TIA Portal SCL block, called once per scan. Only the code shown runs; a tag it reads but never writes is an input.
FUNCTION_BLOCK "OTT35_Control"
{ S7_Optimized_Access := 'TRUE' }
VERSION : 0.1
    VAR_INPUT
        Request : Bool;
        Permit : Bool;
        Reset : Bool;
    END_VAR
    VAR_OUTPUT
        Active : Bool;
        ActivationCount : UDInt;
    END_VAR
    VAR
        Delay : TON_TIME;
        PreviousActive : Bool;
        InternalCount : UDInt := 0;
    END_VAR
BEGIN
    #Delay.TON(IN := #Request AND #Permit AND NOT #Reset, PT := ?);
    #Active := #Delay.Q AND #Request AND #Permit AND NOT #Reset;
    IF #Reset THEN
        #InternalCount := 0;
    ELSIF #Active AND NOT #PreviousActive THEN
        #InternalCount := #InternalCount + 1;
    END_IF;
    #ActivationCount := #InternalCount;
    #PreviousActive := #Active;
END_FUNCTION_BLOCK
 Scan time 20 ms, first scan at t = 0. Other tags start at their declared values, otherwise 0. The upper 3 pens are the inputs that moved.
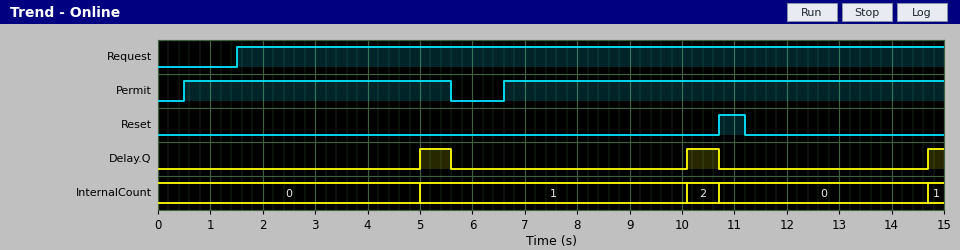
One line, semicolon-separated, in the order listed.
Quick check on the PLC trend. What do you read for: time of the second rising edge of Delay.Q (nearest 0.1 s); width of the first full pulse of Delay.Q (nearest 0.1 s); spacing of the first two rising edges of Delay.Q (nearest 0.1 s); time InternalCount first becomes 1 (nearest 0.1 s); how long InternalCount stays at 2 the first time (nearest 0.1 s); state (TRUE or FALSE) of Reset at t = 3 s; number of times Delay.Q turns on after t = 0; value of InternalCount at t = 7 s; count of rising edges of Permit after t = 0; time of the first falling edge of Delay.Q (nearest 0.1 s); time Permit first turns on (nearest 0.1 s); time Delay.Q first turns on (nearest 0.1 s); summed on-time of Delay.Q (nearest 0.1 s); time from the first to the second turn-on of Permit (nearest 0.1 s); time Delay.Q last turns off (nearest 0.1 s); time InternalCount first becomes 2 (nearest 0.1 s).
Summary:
10.1 s; 0.6 s; 5.1 s; 5.0 s; 0.6 s; FALSE; 3; 1; 2; 5.6 s; 0.5 s; 5.0 s; 1.5 s; 6.1 s; 10.7 s; 10.1 s
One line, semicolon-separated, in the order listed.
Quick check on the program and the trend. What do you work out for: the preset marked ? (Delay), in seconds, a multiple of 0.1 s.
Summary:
3.5 s
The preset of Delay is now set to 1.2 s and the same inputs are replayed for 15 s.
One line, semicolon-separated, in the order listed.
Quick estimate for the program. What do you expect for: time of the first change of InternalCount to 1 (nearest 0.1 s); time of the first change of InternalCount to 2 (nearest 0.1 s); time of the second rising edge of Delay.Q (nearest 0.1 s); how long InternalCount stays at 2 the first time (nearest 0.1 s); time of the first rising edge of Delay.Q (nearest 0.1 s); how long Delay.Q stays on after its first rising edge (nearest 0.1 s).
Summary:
2.7 s; 7.8 s; 7.8 s; 2.9 s; 2.7 s; 2.9 s
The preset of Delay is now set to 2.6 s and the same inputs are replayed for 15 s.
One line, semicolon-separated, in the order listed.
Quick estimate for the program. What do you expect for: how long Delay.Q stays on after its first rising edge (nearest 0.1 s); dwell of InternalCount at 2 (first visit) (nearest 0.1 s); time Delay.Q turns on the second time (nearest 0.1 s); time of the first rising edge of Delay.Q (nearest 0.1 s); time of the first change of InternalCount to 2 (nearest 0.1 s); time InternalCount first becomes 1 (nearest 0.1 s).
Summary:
1.5 s; 1.5 s; 9.2 s; 4.1 s; 9.2 s; 4.1 s
